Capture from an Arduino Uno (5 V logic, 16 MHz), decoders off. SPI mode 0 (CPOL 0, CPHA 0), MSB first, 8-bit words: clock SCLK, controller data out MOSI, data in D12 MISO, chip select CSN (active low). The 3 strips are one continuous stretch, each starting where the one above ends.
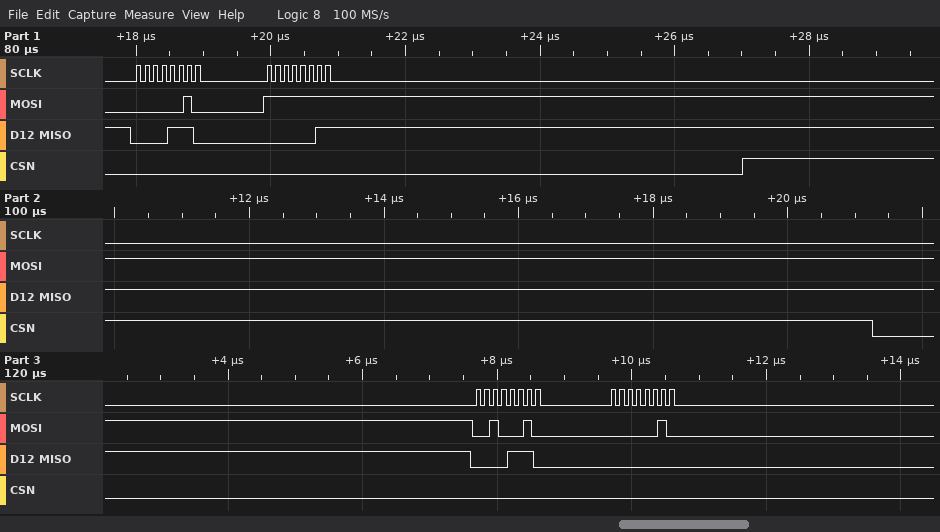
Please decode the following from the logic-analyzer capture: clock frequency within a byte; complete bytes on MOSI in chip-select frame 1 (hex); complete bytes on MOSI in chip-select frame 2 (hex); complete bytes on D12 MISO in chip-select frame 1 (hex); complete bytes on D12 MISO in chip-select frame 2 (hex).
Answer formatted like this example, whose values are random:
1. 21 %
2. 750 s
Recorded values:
1. 8 MHz
2. 02 FF
3. 22 02
4. 0E 03
5. 0E 00
